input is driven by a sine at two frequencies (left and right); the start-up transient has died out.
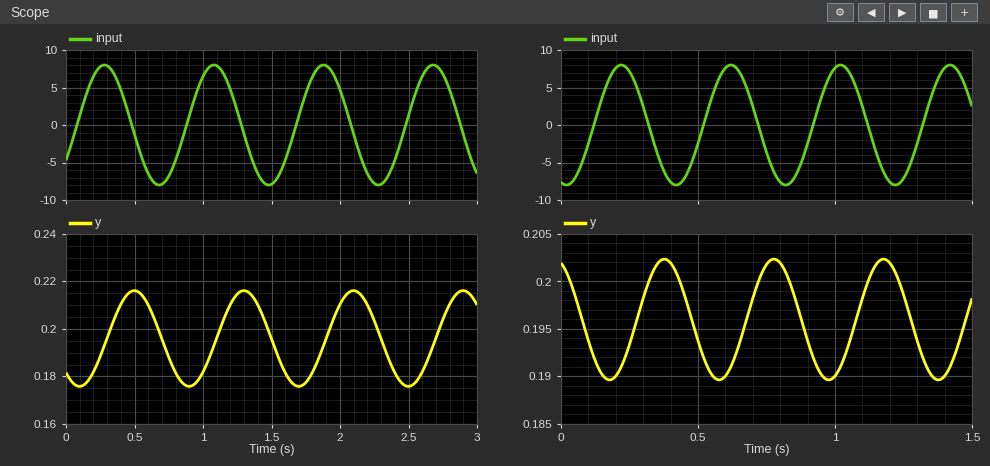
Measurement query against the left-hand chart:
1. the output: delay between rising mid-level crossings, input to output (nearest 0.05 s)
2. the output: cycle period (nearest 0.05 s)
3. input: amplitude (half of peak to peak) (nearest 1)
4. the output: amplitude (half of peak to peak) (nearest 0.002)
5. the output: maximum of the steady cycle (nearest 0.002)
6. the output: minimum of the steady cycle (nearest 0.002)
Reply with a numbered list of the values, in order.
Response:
1. 0.20 s
2. 0.80 s
3. 8
4. 0.020
5. 0.216
6. 0.176
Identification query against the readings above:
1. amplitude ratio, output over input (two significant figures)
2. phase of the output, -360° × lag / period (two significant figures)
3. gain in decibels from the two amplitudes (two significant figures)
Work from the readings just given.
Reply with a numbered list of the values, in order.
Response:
1. 0.0025
2. -90°
3. -52 dB
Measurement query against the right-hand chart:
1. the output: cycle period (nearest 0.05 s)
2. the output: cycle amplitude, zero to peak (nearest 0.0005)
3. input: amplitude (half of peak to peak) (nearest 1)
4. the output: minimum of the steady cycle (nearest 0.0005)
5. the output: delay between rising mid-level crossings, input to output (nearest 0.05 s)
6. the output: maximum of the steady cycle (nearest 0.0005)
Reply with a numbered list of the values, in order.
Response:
1. 0.40 s
2. 0.0065
3. 8
4. 0.1895
5. 0.15 s
6. 0.2025
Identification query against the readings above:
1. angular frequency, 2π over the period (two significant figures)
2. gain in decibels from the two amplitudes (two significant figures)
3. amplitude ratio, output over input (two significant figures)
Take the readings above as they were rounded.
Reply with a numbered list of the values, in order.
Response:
1. 16 rad/s
2. -62 dB
3. 0.00081
